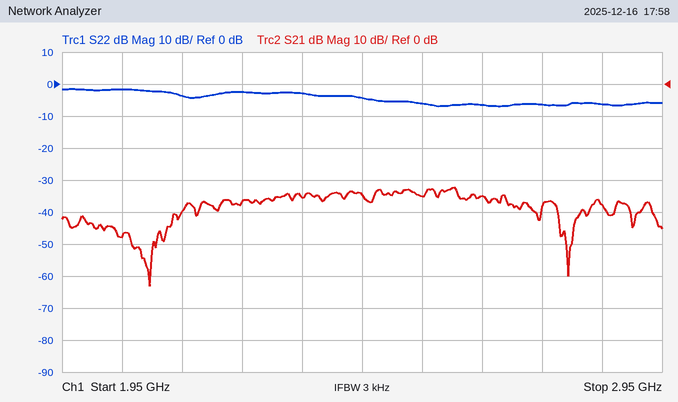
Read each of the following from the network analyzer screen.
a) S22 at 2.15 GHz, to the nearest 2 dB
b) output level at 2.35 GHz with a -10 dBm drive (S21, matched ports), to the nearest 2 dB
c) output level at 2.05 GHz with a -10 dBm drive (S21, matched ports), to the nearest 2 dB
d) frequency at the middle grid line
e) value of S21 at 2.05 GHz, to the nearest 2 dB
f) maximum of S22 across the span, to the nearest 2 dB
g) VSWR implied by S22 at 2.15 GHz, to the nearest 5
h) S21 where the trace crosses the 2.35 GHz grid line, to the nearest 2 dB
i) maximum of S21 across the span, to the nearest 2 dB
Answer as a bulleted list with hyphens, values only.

- -4 dB
- -46 dBm
- -58 dBm
- 2.45 GHz
- -48 dB
- -2 dB
- 5
- -36 dB
- -32 dB
